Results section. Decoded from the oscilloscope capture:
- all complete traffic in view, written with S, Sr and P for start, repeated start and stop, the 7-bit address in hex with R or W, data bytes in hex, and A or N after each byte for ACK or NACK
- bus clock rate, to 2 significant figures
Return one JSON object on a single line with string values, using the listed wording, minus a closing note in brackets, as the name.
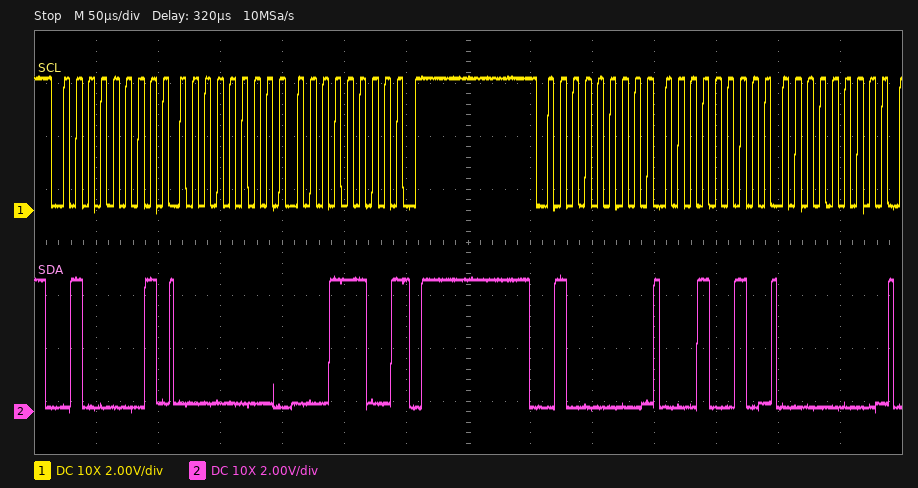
{"all complete traffic in view, written with S, Sr and P for start, repeated start and stop, the 7-bit address in hex with R or W, data bytes in hex, and A or N after each byte for ACK or NACK": "S 20R A 00 A 1C N P S 20W A 12 A 00 A", "bus clock rate, to 2 significant figures": "100 kHz"}
